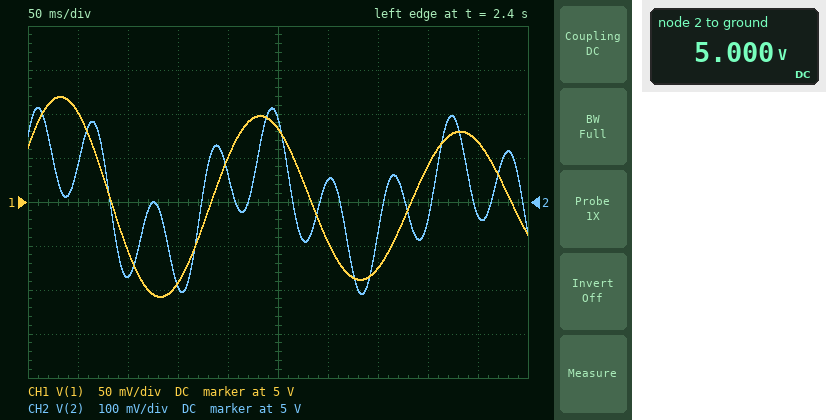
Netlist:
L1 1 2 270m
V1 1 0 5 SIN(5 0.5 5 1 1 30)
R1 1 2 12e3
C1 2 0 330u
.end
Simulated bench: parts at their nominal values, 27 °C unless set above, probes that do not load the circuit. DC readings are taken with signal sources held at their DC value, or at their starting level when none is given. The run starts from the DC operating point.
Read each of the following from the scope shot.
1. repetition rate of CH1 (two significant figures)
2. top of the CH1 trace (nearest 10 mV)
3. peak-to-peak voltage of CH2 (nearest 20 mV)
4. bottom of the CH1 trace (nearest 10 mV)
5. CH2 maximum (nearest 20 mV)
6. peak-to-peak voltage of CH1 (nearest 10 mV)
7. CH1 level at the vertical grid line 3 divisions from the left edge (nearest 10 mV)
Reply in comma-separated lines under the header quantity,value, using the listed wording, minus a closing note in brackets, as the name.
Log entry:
quantity,value
repetition rate of CH1,5.0 Hz
top of the CH1 trace,5.12 V
peak-to-peak voltage of CH2,420 mV
bottom of the CH1 trace,4.89 V
CH2 maximum,5.22 V
peak-to-peak voltage of CH1,230 mV
CH1 level at the vertical grid line 3 divisions from the left edge,4.91 V
